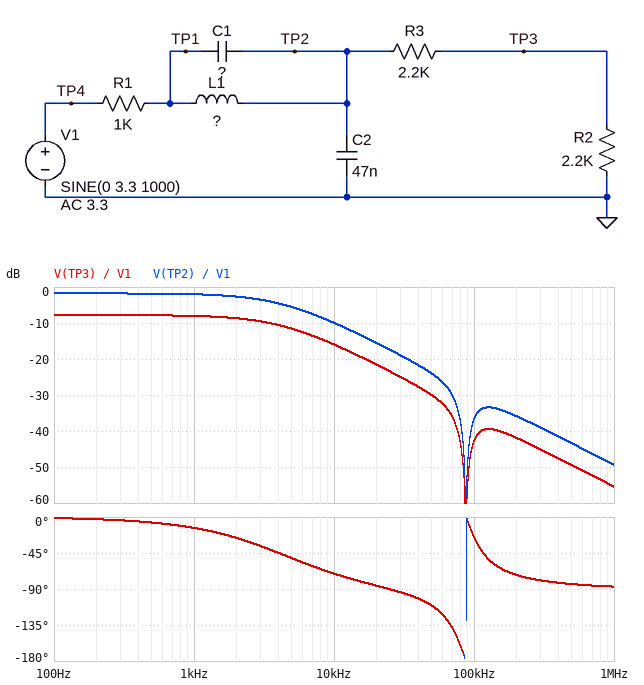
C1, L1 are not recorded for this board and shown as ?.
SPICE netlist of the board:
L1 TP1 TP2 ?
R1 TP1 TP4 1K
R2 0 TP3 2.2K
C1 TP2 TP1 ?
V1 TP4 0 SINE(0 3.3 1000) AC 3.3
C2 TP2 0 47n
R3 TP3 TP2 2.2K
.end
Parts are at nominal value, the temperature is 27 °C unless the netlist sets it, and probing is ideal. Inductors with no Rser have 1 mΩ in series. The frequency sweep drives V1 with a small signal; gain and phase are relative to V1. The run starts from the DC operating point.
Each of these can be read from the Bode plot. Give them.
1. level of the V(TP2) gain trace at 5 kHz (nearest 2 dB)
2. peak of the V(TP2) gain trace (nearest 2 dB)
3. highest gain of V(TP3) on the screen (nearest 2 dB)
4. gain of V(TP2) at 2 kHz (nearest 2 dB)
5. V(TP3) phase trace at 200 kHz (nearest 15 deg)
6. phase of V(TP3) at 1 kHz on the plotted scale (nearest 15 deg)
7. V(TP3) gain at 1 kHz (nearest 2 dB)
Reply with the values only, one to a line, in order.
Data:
-6 dB
-2 dB
-8 dB
-2 dB
-75 deg
-15 deg
-8 dB
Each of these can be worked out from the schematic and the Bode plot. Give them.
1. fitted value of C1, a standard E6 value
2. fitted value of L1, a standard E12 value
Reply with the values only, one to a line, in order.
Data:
3.3 nF
1 mH
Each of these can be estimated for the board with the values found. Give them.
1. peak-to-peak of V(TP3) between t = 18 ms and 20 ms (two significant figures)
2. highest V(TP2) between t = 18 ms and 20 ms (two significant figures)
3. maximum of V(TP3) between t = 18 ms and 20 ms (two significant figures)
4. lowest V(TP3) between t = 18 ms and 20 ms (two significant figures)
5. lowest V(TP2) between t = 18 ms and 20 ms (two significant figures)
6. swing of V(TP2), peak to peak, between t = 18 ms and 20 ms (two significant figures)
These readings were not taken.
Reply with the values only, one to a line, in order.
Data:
2.6 V
2.6 V
1.3 V
-1.3 V
-2.6 V
5.2 V
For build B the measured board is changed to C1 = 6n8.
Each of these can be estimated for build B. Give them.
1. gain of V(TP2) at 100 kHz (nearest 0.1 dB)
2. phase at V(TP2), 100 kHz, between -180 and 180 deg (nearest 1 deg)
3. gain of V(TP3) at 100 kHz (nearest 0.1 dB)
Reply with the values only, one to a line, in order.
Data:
-30.1 dB
-67 deg
-36.1 dB
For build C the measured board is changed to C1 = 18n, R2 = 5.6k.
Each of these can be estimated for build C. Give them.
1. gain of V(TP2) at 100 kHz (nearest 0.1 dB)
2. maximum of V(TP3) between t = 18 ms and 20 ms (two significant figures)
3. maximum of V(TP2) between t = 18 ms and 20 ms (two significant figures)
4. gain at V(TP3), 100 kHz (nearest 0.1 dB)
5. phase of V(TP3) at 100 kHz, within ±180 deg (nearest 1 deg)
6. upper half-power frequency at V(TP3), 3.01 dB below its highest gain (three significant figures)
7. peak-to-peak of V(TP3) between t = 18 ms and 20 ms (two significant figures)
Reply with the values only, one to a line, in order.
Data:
-29.5 dB
2.0 V
2.8 V
-32.4 dB
-82 deg
3.90 kHz
4.1 V
